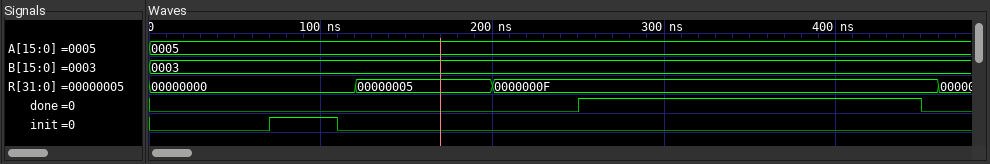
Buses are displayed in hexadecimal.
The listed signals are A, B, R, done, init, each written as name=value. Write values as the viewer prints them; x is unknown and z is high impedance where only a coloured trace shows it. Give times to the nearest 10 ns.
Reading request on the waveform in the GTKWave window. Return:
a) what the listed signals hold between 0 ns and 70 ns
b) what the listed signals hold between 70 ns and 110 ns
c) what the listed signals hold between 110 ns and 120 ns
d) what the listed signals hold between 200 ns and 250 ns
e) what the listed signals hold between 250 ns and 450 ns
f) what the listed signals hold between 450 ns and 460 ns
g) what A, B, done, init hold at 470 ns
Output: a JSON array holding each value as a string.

["A=0005, B=0003, R=00000000, done=0, init=0", "A=0005, B=0003, R=00000000, done=0, init=1", "A=0005, B=0003, R=00000000, done=0, init=0", "A=0005, B=0003, R=0000000F, done=0, init=0", "A=0005, B=0003, R=0000000F, done=1, init=0", "A=0005, B=0003, R=0000000F, done=0, init=0", "A=0005, B=0003, done=0, init=0"]
